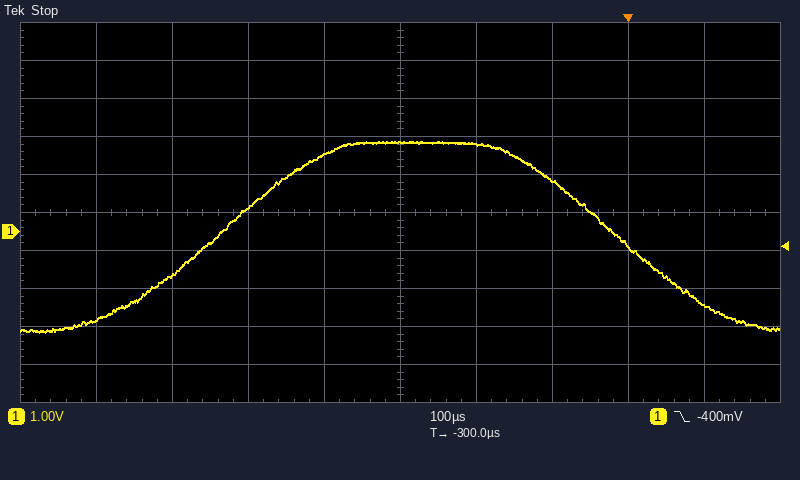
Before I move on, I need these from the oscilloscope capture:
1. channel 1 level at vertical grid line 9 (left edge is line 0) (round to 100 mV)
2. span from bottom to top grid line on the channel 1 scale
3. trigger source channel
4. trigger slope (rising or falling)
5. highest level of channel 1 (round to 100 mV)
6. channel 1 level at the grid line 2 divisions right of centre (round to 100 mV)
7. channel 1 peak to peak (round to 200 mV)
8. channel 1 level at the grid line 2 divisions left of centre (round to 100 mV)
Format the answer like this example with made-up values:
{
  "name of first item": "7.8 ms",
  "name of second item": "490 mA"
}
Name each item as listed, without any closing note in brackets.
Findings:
{
  "channel 1 level at vertical grid line 9 (left edge is line 0)": "-1.9 V",
  "span from bottom to top grid line on the channel 1 scale": "10 V",
  "trigger source channel": "channel 1",
  "trigger slope": "falling",
  "highest level of channel 1": "2.4 V",
  "channel 1 level at the grid line 2 divisions right of centre": "1.4 V",
  "channel 1 peak to peak": "5.0 V",
  "channel 1 level at the grid line 2 divisions left of centre": "600 mV"
}
